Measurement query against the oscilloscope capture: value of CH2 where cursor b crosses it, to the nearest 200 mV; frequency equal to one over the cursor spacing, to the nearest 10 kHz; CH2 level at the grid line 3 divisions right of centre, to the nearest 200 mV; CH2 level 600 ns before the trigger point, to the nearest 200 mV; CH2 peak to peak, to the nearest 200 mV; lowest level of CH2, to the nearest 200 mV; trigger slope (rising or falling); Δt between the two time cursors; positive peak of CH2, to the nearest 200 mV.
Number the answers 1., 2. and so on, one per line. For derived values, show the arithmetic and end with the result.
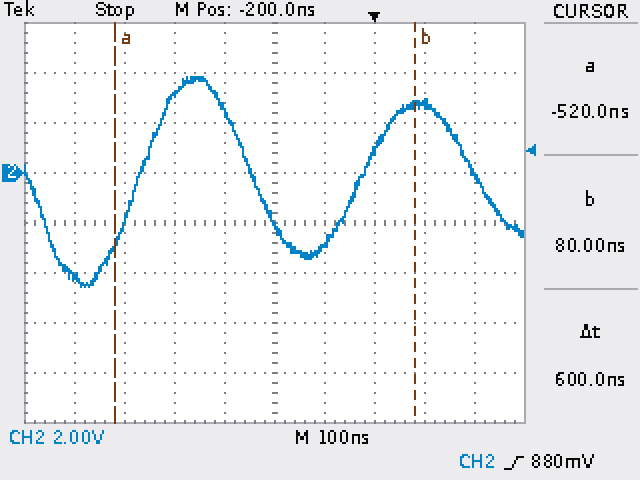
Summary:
1. 2.8 V
2. 1 / 600 ns ≈ 1.67 MHz
3. 2.8 V
4. -4.2 V
5. 3.8 V − (-4.6 V) = 8.4 V
6. -4.6 V
7. rising
8. 600 ns
9. 3.8 V
